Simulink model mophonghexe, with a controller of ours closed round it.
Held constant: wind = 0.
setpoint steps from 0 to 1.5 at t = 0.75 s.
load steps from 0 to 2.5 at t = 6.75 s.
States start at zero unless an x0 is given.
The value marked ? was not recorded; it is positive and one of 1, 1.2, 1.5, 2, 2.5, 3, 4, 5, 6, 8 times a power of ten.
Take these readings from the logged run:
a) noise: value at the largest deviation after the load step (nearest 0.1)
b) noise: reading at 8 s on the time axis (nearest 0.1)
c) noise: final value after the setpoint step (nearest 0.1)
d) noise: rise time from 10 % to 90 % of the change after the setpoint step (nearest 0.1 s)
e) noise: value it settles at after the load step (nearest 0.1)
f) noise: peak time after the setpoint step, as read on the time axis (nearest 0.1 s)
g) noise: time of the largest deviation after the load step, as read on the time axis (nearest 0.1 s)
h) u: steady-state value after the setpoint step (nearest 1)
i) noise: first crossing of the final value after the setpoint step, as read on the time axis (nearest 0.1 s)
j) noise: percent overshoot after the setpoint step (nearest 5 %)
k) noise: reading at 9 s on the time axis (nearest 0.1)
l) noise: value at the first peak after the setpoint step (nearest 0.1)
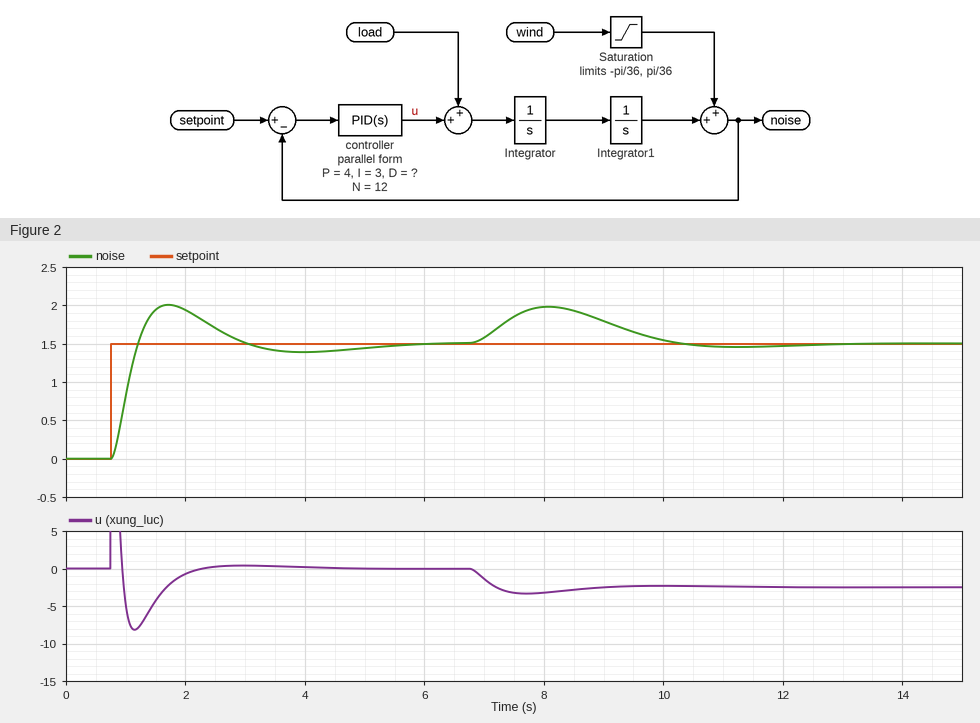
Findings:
2.0
2.0
1.5
0.3 s
1.5
1.7 s
8.1 s
0
1.2 s
35 %
1.8
2.0
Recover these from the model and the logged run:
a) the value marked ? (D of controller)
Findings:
3
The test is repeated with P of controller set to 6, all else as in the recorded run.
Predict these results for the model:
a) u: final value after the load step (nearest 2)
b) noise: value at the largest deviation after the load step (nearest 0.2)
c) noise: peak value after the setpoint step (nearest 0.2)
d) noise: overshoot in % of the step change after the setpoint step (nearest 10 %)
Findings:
-2
1.8
2.0
40 %
